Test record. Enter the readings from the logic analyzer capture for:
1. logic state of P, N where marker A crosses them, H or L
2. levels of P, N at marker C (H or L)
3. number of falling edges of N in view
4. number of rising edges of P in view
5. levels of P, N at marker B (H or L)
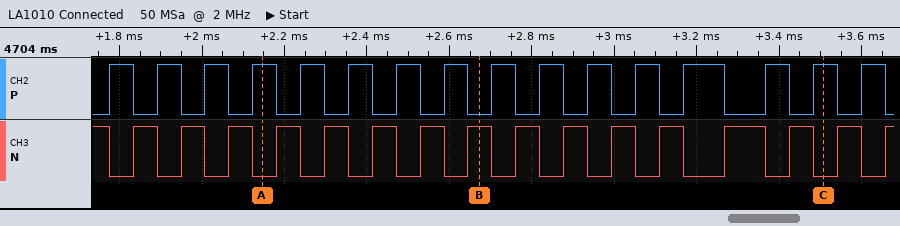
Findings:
P=H, N=L
P=H, N=L
16
16
P=L, N=H
